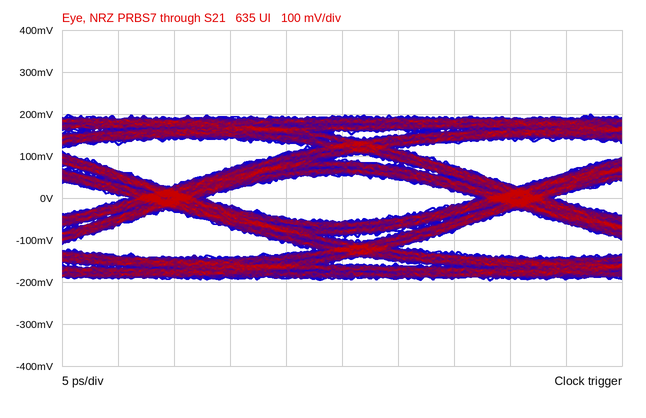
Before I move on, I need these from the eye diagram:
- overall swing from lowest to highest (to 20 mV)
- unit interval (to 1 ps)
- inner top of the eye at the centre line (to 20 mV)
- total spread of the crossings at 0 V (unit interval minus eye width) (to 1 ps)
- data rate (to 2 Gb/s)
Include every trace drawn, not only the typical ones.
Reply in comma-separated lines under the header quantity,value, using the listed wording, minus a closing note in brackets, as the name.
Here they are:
quantity,value
overall swing from lowest to highest,400 mV
unit interval,31 ps
inner top of the eye at the centre line,60 mV
total spread of the crossings at 0 V (unit interval minus eye width),7 ps
data rate,32 Gb/s
